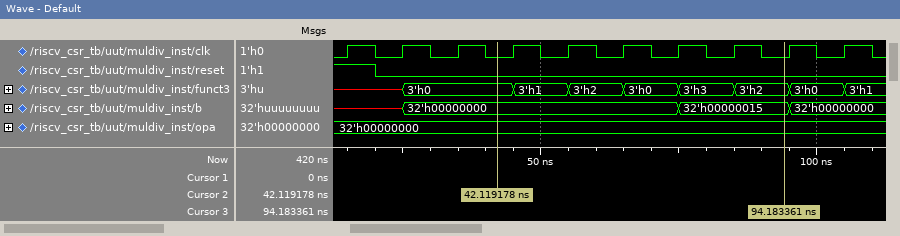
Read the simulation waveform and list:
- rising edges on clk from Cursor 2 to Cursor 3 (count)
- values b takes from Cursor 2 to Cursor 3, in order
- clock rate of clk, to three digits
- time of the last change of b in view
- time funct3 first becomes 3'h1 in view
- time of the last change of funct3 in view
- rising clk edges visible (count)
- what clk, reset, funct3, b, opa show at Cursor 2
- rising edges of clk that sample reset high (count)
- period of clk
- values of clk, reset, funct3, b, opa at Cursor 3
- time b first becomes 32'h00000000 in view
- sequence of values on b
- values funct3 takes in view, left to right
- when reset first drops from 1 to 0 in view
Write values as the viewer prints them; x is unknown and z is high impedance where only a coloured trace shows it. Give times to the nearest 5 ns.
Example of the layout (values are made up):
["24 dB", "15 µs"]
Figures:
["5", "32'h00000000, 32'h00000015", "100 MHz", "95 ns", "45 ns", "105 ns", "10", "clk=0, reset=0, funct3=3'h0, b=32'h00000000, opa=32'h00000000", "1", "10 ns", "clk=0, reset=0, funct3=3'h2, b=32'h00000015, opa=32'h00000000", "25 ns", "x, 32'h00000000, 32'h00000015, 32'h00000000", "x, 3'h0, 3'h1, 3'h2, 3'h0, 3'h3, 3'h2, 3'h0, 3'h1", "20 ns"]
